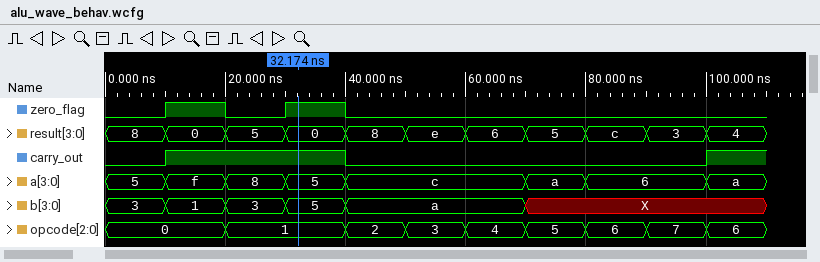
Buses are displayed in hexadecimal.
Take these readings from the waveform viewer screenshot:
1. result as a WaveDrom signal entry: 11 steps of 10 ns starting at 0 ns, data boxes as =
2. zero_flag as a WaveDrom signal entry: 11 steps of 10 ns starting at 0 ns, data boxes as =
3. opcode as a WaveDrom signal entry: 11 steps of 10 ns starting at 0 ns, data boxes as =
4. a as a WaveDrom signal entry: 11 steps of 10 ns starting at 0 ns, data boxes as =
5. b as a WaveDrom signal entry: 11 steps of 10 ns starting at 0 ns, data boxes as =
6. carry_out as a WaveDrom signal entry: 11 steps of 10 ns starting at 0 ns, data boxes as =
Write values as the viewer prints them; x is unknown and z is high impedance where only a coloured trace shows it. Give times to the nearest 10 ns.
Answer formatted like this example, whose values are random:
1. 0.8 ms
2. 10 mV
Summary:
1. {name: 'result', wave: '===========', data: '8 0 5 0 8 e 6 5 c 3 4'}
2. {name: 'zero_flag', wave: '01010......'}
3. {name: 'opcode', wave: '=.=.=======', data: '0 1 2 3 4 5 6 7 6'}
4. {name: 'a', wave: '=====..==.=', data: '5 f 8 5 c a 6 a'}
5. {name: 'b', wave: '=====..x...', data: '3 1 3 5 a'}
6. {name: 'carry_out', wave: '01..0.....1'}
